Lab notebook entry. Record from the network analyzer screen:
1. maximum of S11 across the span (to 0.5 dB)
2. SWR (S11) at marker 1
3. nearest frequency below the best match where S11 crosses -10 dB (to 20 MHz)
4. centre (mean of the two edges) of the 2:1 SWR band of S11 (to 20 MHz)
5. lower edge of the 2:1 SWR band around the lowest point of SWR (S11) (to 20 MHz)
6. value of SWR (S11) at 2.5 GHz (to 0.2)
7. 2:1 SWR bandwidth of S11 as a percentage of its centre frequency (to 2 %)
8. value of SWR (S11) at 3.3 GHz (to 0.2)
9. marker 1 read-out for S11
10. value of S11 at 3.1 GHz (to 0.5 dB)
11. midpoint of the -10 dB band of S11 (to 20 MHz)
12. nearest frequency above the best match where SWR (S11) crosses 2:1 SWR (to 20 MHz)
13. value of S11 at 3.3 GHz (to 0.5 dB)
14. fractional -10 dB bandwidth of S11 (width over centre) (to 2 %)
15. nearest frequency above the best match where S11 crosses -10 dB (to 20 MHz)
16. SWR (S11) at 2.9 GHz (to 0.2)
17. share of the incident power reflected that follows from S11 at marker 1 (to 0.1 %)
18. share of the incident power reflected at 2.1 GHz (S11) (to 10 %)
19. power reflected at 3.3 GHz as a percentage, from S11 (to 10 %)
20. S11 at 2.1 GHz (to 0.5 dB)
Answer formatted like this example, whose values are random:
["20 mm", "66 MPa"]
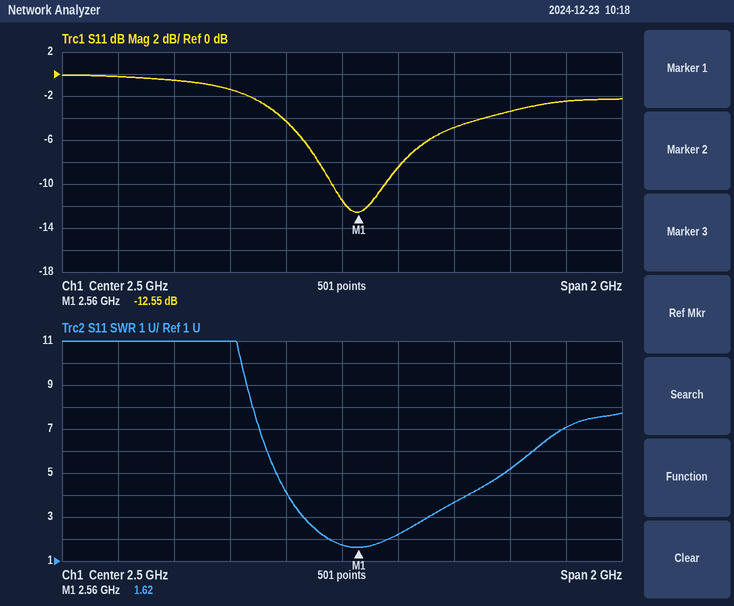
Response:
["0.0 dB", "1.62", "2.46 GHz", "2.56 GHz", "2.46 GHz", "1.8", "8 %", "7.0", "-12.55 dB", "-3.5 dB", "2.56 GHz", "2.66 GHz", "-2.5 dB", "8 %", "2.66 GHz", "3.6", "5.6 %", "70 %", "60 %", "-1.5 dB"]
